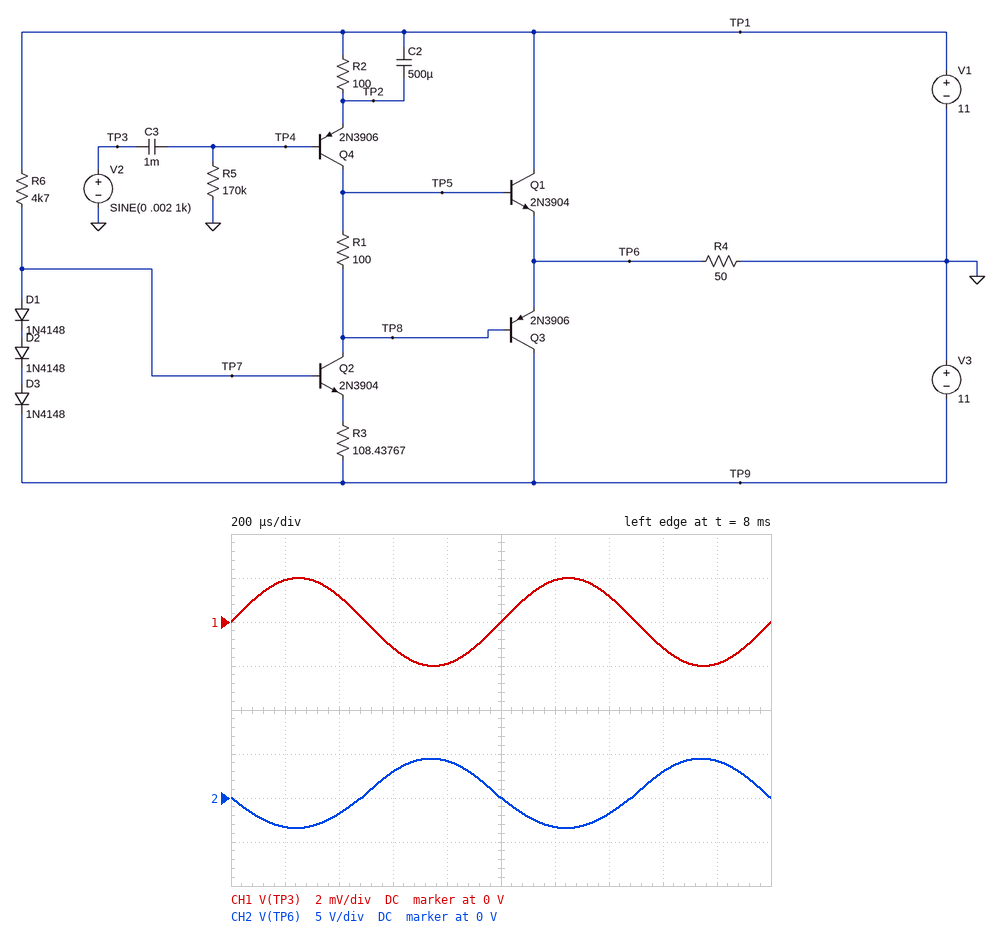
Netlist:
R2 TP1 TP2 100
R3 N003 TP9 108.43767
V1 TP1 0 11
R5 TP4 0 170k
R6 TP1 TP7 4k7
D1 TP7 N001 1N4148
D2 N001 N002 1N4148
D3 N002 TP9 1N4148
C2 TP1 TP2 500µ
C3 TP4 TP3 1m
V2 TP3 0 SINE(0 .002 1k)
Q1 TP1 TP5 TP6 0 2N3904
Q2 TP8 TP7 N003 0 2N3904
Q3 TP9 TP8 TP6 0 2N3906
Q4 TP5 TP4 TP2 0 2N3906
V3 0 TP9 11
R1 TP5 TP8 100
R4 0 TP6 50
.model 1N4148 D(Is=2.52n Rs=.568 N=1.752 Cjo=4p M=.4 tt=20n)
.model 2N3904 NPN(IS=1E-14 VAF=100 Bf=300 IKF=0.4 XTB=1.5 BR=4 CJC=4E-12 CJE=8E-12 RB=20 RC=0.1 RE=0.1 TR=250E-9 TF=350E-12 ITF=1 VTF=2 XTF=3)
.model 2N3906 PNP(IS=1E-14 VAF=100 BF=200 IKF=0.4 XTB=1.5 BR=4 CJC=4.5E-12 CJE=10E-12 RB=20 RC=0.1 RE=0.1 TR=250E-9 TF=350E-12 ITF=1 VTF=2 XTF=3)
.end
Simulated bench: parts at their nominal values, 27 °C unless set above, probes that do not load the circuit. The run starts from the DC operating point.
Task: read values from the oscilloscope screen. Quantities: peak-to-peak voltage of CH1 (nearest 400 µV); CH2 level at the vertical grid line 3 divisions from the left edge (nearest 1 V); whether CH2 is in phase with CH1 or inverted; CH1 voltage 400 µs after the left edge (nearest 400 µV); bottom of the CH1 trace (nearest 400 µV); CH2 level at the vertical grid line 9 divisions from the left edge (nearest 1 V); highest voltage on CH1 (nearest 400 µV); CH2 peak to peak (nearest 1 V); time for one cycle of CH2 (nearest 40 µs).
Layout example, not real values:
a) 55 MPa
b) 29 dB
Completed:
a) 4.0 mV
b) 3 V
c) inverted
d) 1.2 mV
e) -2.0 mV
f) 4 V
g) 2.0 mV
h) 8 V
i) 1.00 ms
